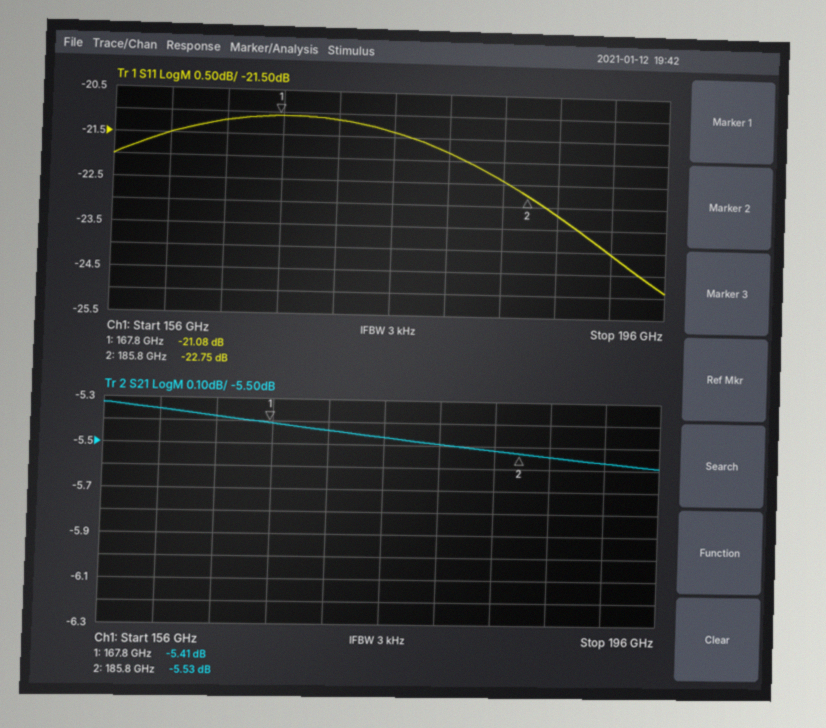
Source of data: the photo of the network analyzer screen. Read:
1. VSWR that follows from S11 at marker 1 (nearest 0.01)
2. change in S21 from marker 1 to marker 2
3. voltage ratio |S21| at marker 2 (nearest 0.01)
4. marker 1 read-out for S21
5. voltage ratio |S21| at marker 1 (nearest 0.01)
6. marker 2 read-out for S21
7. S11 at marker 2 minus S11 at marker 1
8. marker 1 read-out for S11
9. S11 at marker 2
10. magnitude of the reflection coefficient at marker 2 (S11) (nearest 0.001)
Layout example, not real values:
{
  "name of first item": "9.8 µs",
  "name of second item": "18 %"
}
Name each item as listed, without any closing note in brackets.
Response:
{
  "VSWR that follows from S11 at marker 1": "1.19",
  "change in S21 from marker 1 to marker 2": "-0.12 dB",
  "voltage ratio |S21| at marker 2": "0.53",
  "marker 1 read-out for S21": "-5.41 dB",
  "voltage ratio |S21| at marker 1": "0.54",
  "marker 2 read-out for S21": "-5.53 dB",
  "S11 at marker 2 minus S11 at marker 1": "-1.67 dB",
  "marker 1 read-out for S11": "-21.08 dB",
  "S11 at marker 2": "-22.75 dB",
  "magnitude of the reflection coefficient at marker 2 (S11)": "0.073"
}
